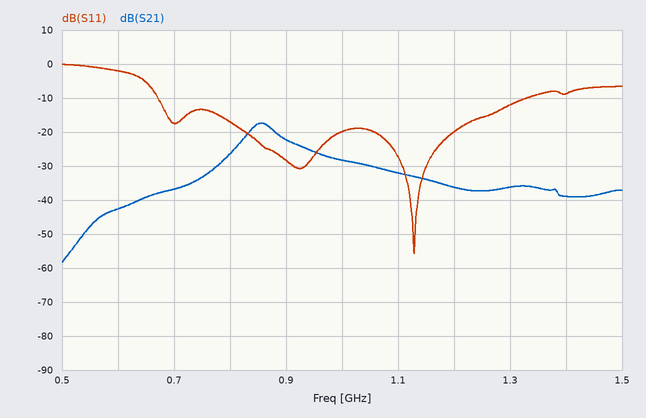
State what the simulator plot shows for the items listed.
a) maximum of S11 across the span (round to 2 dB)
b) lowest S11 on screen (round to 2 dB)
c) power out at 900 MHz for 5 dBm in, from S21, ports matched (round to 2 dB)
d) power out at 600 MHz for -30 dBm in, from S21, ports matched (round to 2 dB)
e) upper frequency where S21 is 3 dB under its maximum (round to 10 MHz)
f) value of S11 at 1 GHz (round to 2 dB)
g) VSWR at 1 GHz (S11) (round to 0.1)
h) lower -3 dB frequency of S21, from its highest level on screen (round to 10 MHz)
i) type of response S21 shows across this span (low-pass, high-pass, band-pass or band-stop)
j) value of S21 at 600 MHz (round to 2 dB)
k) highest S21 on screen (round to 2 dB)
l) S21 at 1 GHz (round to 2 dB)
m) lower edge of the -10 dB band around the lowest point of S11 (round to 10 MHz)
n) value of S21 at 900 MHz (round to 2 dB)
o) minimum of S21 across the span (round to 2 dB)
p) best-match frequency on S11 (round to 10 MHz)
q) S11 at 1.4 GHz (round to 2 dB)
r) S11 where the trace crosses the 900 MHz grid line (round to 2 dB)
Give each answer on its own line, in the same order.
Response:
0 dB
-56 dB
-18 dBm
-72 dBm
880 MHz
-20 dB
1.2
830 MHz
band-pass
-42 dB
-18 dB
-28 dB
670 MHz
-22 dB
-58 dB
1.13 GHz
-8 dB
-28 dB
